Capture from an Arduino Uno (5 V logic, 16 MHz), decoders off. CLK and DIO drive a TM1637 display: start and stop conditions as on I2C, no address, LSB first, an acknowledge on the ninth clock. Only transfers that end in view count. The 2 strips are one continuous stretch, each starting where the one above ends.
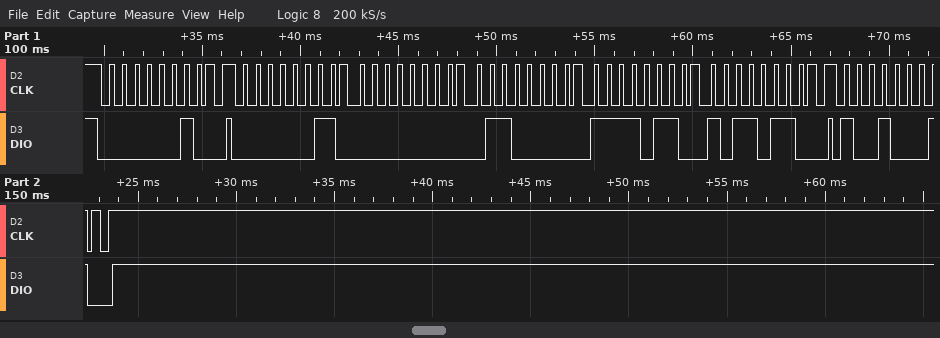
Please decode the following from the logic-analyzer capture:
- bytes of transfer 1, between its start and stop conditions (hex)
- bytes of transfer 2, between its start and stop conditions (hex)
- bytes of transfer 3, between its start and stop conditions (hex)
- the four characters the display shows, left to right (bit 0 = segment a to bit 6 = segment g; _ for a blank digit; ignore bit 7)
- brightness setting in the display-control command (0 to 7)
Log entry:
40
C0 00 06 6F 6D
89
_195
1
